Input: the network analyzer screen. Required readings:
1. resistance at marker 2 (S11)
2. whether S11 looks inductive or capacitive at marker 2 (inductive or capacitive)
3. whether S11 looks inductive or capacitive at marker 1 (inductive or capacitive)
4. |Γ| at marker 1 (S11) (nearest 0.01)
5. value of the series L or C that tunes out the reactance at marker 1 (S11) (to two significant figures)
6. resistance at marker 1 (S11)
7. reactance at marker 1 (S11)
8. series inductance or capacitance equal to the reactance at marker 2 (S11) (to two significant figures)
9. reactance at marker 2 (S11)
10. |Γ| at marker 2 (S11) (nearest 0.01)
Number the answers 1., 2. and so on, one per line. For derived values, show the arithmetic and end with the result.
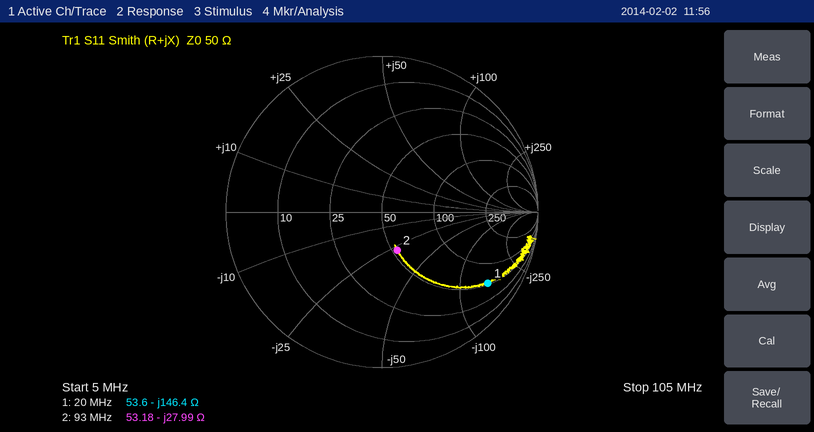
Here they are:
1. 53.18 Ω
2. capacitive
3. capacitive
4. 0.82
5. L = 146.4 Ω/(2π × 20 MHz) ≈ 1.2 µH
6. 53.6 Ω
7. -146.4 Ω
8. C = 1/(2π × 93 MHz × 27.99 Ω) ≈ 61 pF
9. -27.99 Ω
10. 0.26
